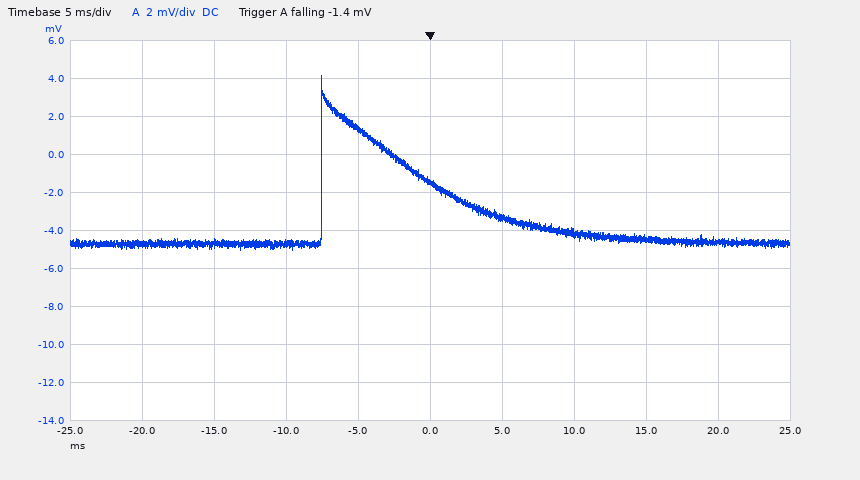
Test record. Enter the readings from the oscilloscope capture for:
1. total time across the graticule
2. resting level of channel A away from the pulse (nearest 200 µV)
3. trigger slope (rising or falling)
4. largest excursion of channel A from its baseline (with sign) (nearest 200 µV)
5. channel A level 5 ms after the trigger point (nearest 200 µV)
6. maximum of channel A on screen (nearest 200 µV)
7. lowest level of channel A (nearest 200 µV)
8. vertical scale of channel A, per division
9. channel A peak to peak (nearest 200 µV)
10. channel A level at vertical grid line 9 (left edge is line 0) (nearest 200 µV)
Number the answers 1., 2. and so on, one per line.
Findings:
1. 50 ms
2. -4.6 mV
3. falling
4. +8.8 mV
5. -3.2 mV
6. 4.2 mV
7. -5.0 mV
8. 2 mV
9. 9.2 mV
10. -4.6 mV
